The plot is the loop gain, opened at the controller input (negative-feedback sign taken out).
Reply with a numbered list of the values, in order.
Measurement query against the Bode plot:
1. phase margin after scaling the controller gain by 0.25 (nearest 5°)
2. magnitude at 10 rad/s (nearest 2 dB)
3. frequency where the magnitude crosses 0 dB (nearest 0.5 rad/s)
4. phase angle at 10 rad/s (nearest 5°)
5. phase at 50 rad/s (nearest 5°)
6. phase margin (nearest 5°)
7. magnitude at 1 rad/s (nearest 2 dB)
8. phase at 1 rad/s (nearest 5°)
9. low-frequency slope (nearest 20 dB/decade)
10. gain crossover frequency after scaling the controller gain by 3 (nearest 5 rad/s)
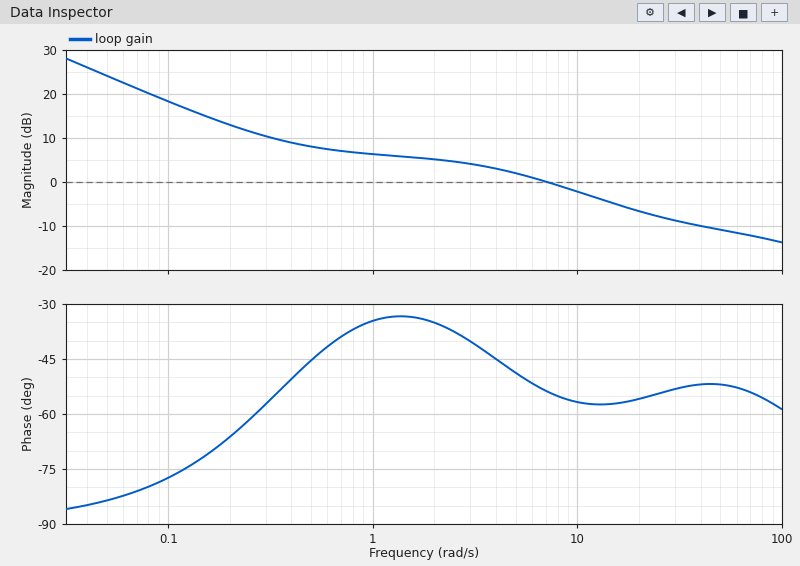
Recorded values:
1. 115°
2. -2 dB
3. 7.0 rad/s
4. -55°
5. -50°
6. 125°
7. 6 dB
8. -35°
9. -20 dB/decade
10. 35 rad/s
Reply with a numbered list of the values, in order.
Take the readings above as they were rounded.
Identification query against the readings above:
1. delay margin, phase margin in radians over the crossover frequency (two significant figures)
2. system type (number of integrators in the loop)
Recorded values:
1. 0.31 s
2. 1
